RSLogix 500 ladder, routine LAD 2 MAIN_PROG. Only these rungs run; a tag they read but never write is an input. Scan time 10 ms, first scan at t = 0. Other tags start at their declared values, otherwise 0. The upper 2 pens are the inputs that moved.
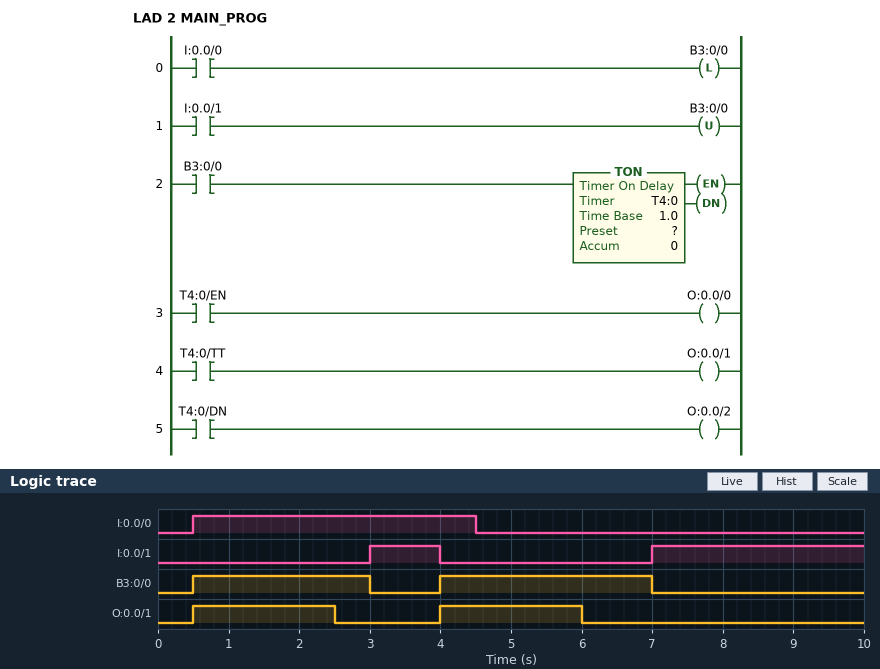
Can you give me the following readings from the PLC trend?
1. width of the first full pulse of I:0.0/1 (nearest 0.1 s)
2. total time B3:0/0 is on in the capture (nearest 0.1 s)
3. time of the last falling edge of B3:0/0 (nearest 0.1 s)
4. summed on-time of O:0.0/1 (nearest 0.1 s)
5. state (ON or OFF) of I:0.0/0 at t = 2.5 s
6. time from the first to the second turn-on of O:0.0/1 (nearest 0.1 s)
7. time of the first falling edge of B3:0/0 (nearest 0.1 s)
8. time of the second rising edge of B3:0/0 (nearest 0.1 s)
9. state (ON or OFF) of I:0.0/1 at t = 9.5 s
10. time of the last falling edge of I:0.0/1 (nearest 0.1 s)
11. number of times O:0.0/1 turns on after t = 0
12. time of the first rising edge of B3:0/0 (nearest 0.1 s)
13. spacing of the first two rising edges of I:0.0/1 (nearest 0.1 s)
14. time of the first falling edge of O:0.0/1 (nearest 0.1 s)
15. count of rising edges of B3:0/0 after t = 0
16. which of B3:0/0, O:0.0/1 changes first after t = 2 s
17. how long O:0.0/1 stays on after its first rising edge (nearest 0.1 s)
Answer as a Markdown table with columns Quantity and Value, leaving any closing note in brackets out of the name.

| Quantity | Value |
|---|---|
| width of the first full pulse of I:0.0/1 | 1.0 s |
| total time B3:0/0 is on in the capture | 5.5 s |
| time of the last falling edge of B3:0/0 | 7.0 s |
| summed on-time of O:0.0/1 | 4.0 s |
| state (ON or OFF) of I:0.0/0 at t = 2.5 s | ON |
| time from the first to the second turn-on of O:0.0/1 | 3.5 s |
| time of the first falling edge of B3:0/0 | 3.0 s |
| time of the second rising edge of B3:0/0 | 4.0 s |
| state (ON or OFF) of I:0.0/1 at t = 9.5 s | ON |
| time of the last falling edge of I:0.0/1 | 4.0 s |
| number of times O:0.0/1 turns on after t = 0 | 2 |
| time of the first rising edge of B3:0/0 | 0.5 s |
| spacing of the first two rising edges of I:0.0/1 | 4.0 s |
| time of the first falling edge of O:0.0/1 | 2.5 s |
| count of rising edges of B3:0/0 after t = 0 | 2 |
| which of B3:0/0, O:0.0/1 changes first after t = 2 s | O:0.0/1 |
| how long O:0.0/1 stays on after its first rising edge | 2.0 s |
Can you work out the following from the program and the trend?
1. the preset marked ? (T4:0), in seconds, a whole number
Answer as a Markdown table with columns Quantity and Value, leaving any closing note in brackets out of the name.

| Quantity | Value |
|---|---|
| the preset marked ? (T4:0), in seconds, a whole number | 2 s |
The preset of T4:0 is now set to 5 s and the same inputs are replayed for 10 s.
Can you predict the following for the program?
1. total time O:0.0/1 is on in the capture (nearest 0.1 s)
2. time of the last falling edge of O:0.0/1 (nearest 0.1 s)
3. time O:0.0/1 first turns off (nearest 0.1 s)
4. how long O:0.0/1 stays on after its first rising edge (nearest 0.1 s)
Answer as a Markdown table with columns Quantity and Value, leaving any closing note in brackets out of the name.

| Quantity | Value |
|---|---|
| total time O:0.0/1 is on in the capture | 5.5 s |
| time of the last falling edge of O:0.0/1 | 7.0 s |
| time O:0.0/1 first turns off | 3.0 s |
| how long O:0.0/1 stays on after its first rising edge | 2.5 s |
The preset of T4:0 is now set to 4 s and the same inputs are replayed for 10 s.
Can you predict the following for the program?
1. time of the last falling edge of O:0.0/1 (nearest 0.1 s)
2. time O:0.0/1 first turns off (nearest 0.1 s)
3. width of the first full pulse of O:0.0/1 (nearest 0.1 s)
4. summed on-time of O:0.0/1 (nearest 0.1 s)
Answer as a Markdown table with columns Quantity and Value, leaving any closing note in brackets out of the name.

| Quantity | Value |
|---|---|
| time of the last falling edge of O:0.0/1 | 7.0 s |
| time O:0.0/1 first turns off | 3.0 s |
| width of the first full pulse of O:0.0/1 | 2.5 s |
| summed on-time of O:0.0/1 | 5.5 s |
